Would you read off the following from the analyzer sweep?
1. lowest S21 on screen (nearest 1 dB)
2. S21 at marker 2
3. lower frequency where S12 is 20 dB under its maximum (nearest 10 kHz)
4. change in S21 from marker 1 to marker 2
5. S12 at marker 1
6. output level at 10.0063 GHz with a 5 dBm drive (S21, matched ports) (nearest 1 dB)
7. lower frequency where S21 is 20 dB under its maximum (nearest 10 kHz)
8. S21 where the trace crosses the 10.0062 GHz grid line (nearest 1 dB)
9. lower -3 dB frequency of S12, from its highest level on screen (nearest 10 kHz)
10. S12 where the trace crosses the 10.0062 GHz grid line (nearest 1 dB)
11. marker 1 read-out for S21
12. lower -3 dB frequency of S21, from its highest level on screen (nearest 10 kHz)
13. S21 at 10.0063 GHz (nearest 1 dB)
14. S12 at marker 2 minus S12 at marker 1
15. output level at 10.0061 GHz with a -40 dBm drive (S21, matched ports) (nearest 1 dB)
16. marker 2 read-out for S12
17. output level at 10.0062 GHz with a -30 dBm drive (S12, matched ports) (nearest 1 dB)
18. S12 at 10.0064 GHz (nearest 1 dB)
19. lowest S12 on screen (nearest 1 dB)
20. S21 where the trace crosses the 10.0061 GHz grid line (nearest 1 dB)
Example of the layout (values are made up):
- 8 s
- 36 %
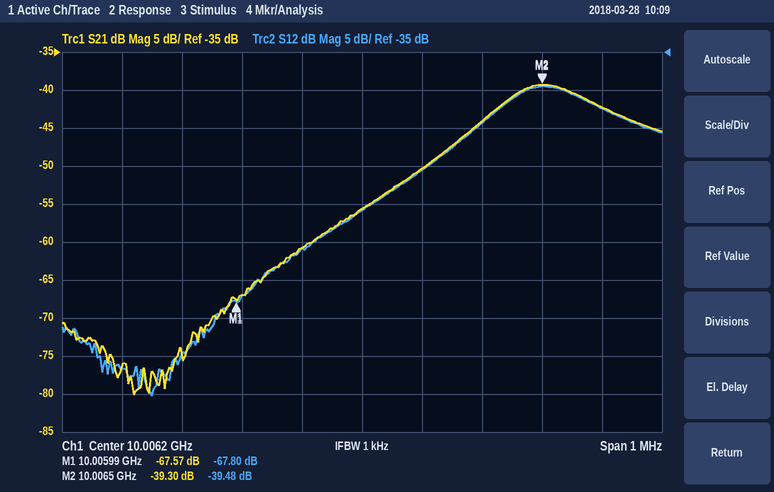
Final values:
- -80 dB
- -39.30 dB
- 10.00613 GHz
- 28.27 dB
- -67.80 dB
- -45 dBm
- 10.00613 GHz
- -56 dB
- 10.00643 GHz
- -56 dB
- -67.57 dB
- 10.00643 GHz
- -50 dB
- 28.32 dB
- -101 dBm
- -39.48 dB
- -86 dBm
- -44 dB
- -80 dB
- -61 dB
